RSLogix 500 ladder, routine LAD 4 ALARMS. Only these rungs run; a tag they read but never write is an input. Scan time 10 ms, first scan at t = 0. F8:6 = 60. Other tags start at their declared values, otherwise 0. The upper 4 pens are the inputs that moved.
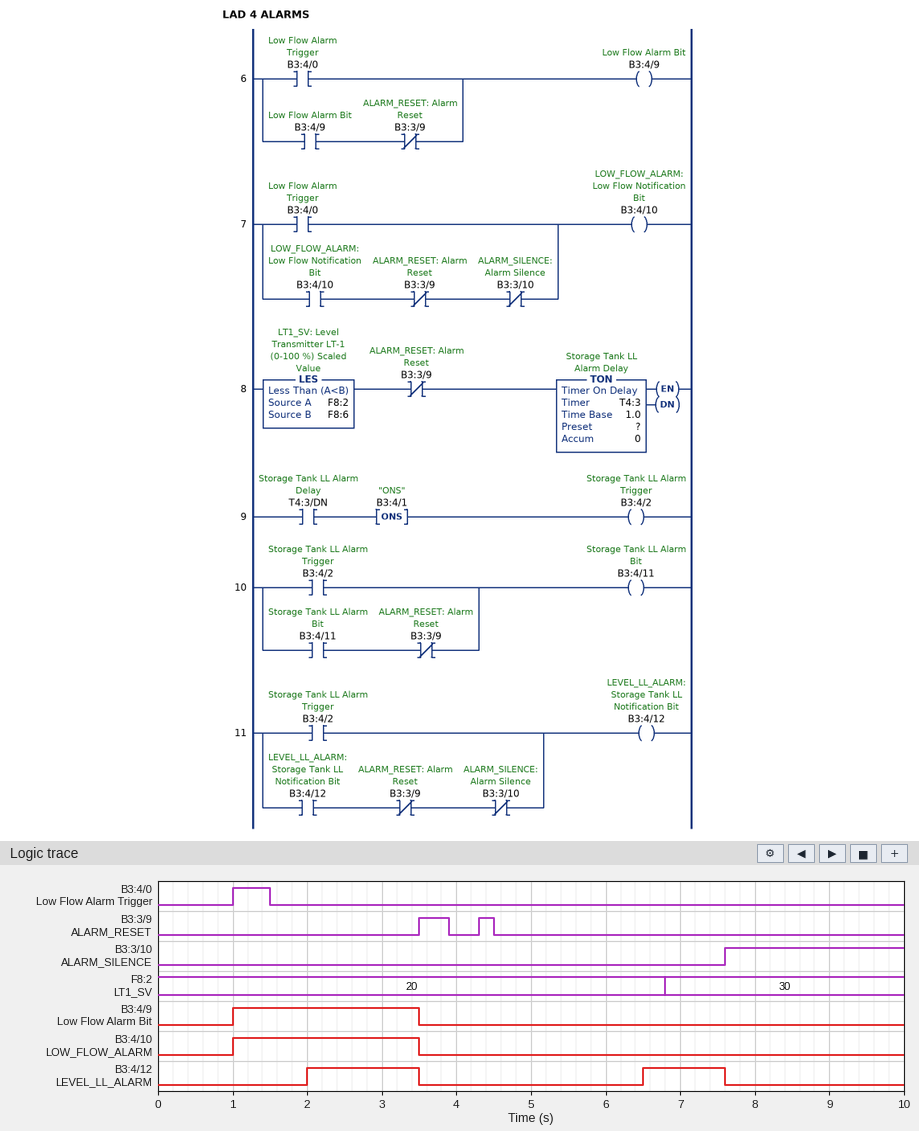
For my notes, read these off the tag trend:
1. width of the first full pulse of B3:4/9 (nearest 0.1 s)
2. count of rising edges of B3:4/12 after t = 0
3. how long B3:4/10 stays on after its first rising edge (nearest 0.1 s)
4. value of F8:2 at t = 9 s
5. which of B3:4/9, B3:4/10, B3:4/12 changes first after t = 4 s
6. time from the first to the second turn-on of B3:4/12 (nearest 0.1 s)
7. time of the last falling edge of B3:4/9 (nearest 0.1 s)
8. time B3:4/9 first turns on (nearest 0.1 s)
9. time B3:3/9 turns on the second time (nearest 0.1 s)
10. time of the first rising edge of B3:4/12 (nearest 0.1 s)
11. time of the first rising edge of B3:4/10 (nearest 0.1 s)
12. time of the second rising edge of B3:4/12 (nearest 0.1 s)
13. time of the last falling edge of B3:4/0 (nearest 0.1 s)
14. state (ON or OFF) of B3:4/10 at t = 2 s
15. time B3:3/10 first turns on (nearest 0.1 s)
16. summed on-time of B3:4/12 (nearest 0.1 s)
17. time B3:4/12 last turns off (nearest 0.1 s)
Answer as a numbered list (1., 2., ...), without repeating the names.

1. 2.5 s
2. 2
3. 2.5 s
4. 30
5. B3:4/12
6. 4.5 s
7. 3.5 s
8. 1.0 s
9. 4.3 s
10. 2.0 s
11. 1.0 s
12. 6.5 s
13. 1.5 s
14. ON
15. 7.6 s
16. 2.6 s
17. 7.6 s
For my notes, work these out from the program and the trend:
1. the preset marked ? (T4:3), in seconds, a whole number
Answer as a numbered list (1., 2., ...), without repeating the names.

1. 2 s
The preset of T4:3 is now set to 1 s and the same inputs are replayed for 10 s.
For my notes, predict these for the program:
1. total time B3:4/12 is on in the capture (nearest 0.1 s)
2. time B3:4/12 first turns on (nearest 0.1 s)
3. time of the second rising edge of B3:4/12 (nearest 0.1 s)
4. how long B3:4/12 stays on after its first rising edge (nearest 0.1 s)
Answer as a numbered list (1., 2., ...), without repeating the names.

1. 4.6 s
2. 1.0 s
3. 5.5 s
4. 2.5 s
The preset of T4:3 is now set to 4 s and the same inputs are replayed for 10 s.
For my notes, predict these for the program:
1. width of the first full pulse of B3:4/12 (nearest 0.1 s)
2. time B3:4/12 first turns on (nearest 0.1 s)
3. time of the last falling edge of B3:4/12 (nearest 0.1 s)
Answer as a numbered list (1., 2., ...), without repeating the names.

1. 0.0 s
2. 8.5 s
3. 8.5 s
